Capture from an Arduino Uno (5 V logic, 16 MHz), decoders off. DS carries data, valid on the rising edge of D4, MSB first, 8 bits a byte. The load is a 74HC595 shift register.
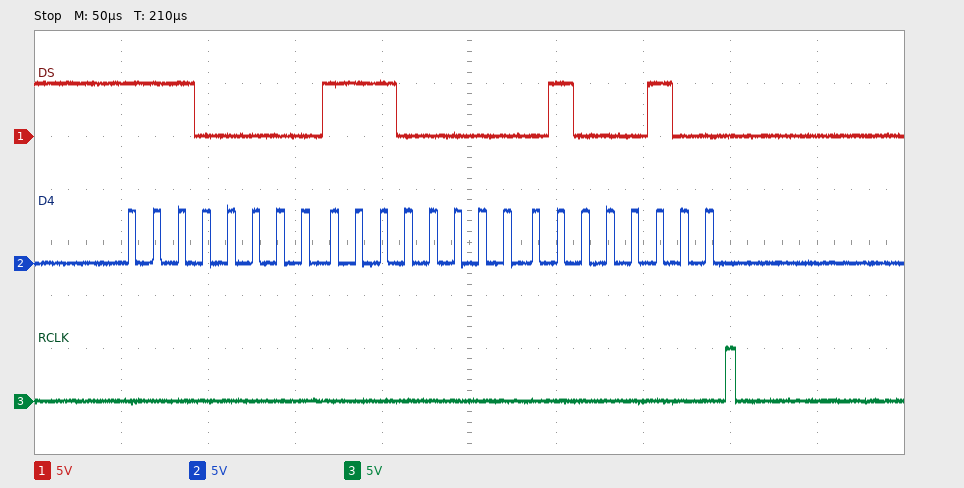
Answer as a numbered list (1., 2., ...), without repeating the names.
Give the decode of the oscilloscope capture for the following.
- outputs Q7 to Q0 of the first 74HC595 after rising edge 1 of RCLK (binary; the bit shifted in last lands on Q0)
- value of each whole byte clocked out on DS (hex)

1. 01000100
2. E0 E0 44
